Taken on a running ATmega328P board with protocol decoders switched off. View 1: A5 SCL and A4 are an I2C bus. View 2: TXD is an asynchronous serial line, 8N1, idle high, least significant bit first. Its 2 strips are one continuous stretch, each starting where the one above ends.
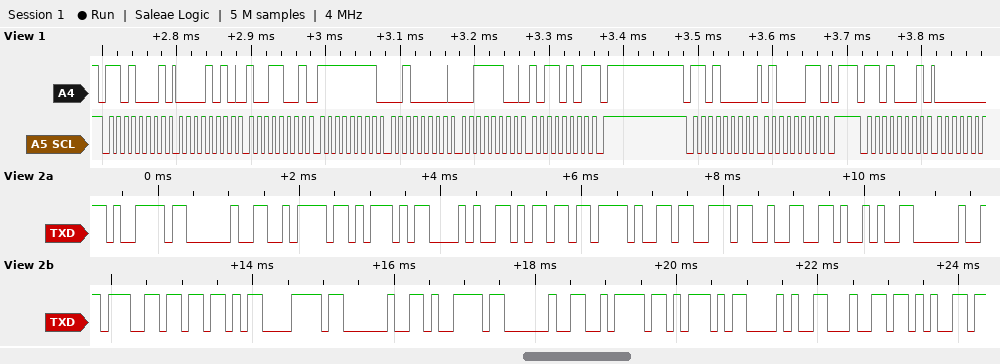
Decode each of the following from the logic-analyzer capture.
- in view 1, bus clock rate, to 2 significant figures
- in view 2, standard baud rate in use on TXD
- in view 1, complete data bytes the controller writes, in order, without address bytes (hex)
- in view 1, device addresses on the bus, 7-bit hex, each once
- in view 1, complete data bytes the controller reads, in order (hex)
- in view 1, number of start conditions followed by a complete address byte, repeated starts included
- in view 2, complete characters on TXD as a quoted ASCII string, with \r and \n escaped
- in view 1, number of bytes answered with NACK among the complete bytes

100 kHz
9600 baud
43
0x68
0A 99 FF 20 3C B5
3
"y z](m/s2) g[x y z](de"
1
